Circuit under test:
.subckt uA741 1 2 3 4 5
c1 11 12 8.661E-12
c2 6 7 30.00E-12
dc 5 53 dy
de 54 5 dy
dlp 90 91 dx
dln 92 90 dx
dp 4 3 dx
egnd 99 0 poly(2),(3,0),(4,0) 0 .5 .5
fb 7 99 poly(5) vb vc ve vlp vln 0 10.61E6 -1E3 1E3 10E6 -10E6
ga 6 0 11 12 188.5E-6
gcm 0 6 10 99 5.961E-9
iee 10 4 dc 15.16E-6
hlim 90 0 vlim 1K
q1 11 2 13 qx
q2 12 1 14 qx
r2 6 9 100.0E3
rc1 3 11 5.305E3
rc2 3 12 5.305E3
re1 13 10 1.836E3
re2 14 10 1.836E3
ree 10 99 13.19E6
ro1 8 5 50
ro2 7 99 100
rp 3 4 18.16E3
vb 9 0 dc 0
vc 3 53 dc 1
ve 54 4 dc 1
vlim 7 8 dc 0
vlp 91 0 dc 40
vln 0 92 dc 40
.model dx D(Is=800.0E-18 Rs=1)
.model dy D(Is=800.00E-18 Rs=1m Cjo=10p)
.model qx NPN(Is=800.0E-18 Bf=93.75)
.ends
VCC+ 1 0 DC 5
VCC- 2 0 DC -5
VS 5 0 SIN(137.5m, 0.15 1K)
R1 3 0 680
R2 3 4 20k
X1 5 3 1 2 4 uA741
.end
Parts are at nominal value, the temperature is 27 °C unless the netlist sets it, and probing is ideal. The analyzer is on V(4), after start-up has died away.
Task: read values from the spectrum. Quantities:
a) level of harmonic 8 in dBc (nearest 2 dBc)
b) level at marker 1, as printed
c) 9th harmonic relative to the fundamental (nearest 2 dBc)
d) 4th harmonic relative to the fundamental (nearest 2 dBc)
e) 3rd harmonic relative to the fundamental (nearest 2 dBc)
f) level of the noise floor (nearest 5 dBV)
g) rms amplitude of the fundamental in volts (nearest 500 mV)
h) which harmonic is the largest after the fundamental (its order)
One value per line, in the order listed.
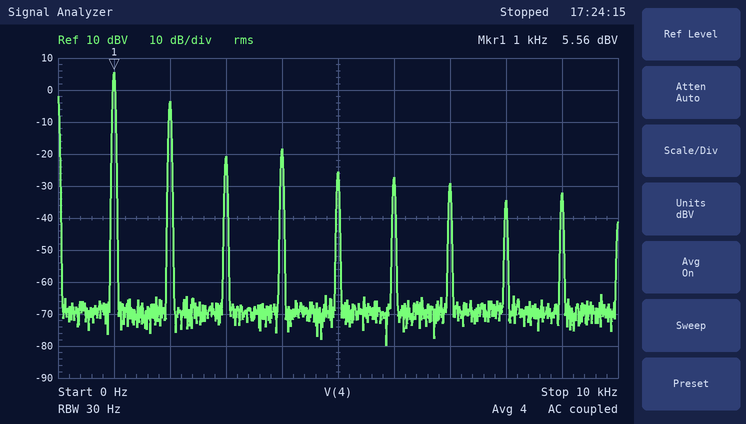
-40 dBc
5.56 dBV
-38 dBc
-24 dBc
-26 dBc
-70 dBV
2.0 V
2
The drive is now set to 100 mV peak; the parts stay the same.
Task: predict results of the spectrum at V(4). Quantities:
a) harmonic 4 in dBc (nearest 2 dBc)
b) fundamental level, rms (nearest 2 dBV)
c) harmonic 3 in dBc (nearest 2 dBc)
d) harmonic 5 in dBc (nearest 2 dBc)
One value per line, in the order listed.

-26 dBc
2 dBV
-24 dBc
-30 dBc
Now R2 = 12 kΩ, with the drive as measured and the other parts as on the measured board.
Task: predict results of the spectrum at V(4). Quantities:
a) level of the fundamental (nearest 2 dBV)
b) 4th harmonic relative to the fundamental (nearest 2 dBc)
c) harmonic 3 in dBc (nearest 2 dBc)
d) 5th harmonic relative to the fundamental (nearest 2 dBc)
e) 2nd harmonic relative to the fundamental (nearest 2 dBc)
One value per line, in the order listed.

6 dBV
-32 dBc
-28 dBc
-36 dBc
-26 dBc
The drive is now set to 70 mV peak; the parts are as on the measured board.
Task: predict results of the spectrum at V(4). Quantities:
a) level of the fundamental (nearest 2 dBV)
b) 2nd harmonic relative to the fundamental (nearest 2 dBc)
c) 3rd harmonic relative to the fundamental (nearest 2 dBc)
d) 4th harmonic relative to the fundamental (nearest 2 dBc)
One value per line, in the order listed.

0 dBV
-12 dBc
-22 dBc
-32 dBc
